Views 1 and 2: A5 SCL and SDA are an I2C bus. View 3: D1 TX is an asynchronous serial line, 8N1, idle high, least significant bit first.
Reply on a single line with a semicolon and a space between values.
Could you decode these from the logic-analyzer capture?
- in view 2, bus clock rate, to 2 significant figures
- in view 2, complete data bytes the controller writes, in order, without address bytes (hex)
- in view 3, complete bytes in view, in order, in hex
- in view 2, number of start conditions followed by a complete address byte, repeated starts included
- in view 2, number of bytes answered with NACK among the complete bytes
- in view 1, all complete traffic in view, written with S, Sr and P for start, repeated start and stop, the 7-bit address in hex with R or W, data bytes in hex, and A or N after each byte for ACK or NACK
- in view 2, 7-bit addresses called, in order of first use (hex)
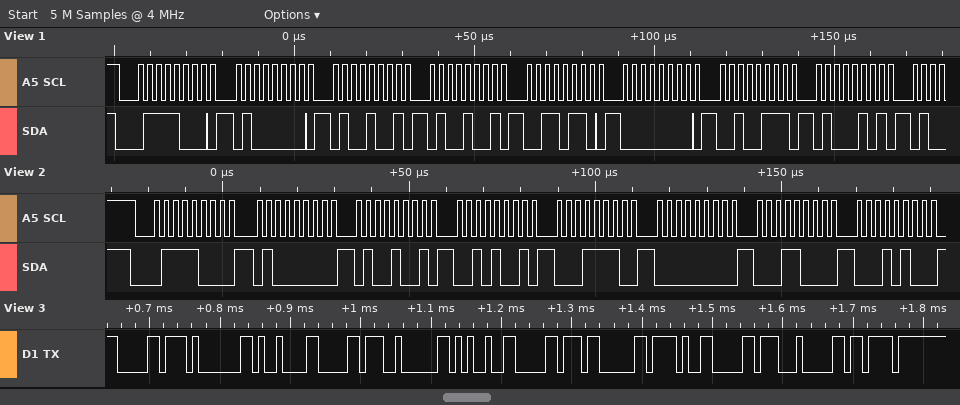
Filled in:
400 kHz; 40 49 29 1E 00 18 14; 0xB0 0x01 0x09 0xB0 0x02 0x25 0xB0 0x03 0x2F 0xB0 0x04 0x7B; 1; 0; S 3CW A 40 A 49 A 49 A 36 A 00 A 27 A 45 A; 0x3C
